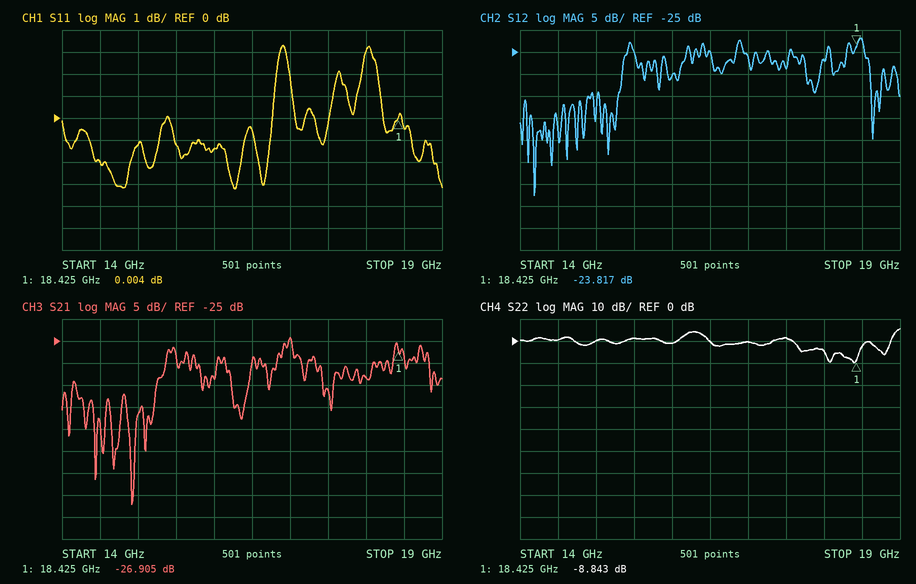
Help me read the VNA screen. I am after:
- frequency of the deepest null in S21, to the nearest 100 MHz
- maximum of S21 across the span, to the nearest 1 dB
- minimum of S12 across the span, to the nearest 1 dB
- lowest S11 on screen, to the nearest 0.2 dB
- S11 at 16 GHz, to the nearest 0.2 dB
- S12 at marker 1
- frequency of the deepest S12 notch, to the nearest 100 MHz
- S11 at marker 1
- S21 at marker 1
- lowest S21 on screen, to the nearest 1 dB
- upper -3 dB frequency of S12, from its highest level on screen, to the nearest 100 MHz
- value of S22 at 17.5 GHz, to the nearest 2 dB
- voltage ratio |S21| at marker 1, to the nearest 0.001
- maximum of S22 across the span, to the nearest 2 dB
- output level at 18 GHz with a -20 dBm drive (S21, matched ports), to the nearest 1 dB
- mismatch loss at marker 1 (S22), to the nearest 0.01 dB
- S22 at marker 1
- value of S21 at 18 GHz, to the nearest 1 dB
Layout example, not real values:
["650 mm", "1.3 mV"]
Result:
["14.9 GHz", "-24 dB", "-58 dB", "-3.2 dB", "-1.4 dB", "-23.817 dB", "14.2 GHz", "0.004 dB", "-26.905 dB", "-62 dB", "18.5 GHz", "2 dB", "0.045", "6 dB", "-53 dBm", "0.61 dB", "-8.843 dB", "-33 dB"]
